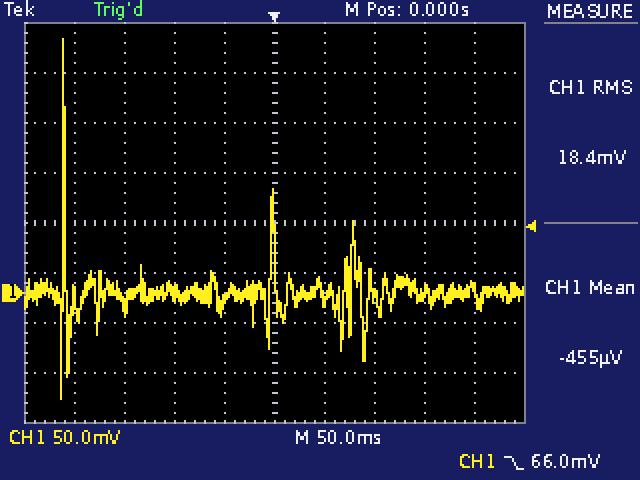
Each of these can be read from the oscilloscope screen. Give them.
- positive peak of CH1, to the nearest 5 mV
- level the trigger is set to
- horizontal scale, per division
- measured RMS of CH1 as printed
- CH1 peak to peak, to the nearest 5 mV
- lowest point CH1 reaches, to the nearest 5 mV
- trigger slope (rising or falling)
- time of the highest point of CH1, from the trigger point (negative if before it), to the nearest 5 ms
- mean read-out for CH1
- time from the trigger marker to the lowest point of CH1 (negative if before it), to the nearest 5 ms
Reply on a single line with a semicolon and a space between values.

255 mV; 66.0 mV; 50 ms; 18.4 mV; 360 mV; -105 mV; falling; -210 ms; -455 µV; -215 ms
